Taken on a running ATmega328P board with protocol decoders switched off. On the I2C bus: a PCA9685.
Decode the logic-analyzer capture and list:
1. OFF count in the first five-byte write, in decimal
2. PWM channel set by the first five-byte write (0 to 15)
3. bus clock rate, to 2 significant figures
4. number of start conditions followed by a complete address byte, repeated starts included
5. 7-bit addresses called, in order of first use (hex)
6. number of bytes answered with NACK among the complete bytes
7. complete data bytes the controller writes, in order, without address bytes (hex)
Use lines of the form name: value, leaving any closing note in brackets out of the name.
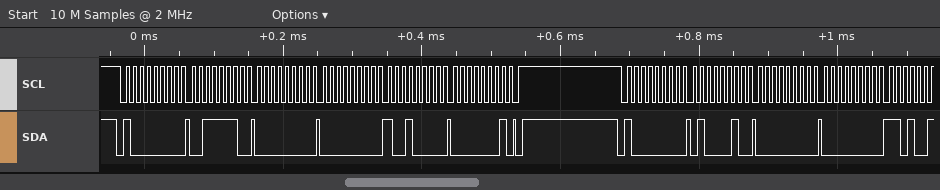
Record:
OFF count in the first five-byte write, in decimal: 400
PWM channel set by the first five-byte write: 14
bus clock rate, to 2 significant figures: 100 kHz
number of start conditions followed by a complete address byte, repeated starts included: 2
7-bit addresses called, in order of first use: 0x40
number of bytes answered with NACK among the complete bytes: 0
complete data bytes the controller writes, in order, without address bytes: 3E 00 00 90 01 42 00 00
